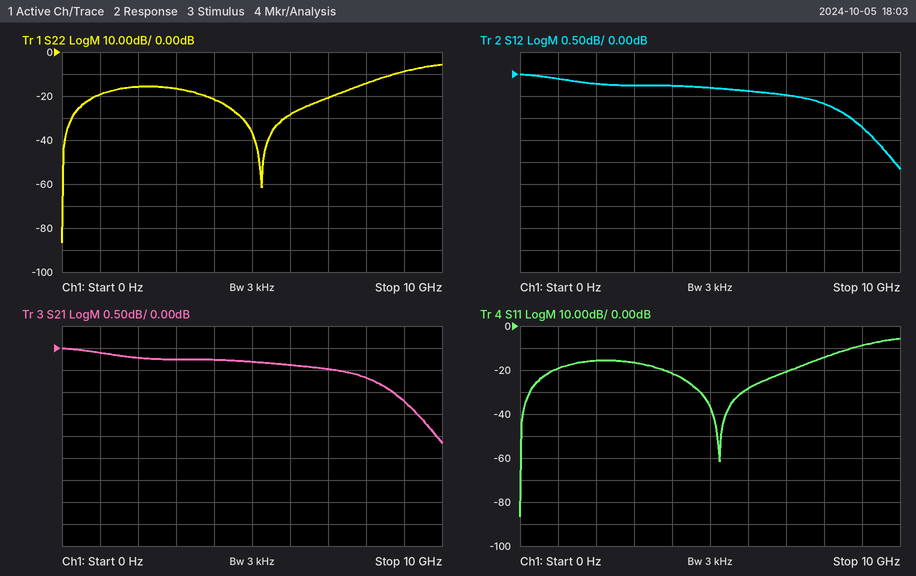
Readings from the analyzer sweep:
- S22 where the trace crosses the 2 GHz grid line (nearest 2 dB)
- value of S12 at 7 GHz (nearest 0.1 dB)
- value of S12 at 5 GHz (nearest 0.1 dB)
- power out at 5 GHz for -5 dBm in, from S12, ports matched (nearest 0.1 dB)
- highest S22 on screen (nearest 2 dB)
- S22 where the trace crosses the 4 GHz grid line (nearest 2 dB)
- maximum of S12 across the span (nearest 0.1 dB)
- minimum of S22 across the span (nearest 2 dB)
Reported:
-16 dB
-0.5 dB
-0.3 dB
-5.3 dBm
-6 dB
-22 dB
0.0 dB
-86 dB
